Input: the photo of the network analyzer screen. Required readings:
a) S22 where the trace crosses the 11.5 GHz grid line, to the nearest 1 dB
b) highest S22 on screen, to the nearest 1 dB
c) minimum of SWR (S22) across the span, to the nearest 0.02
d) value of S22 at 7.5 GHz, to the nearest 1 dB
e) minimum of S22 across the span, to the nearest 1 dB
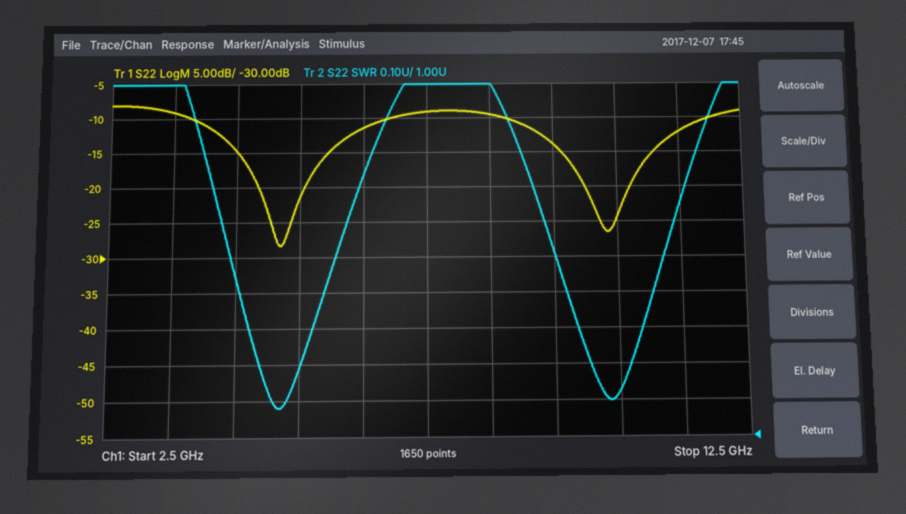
-12 dB
-8 dB
1.08
-9 dB
-28 dB
